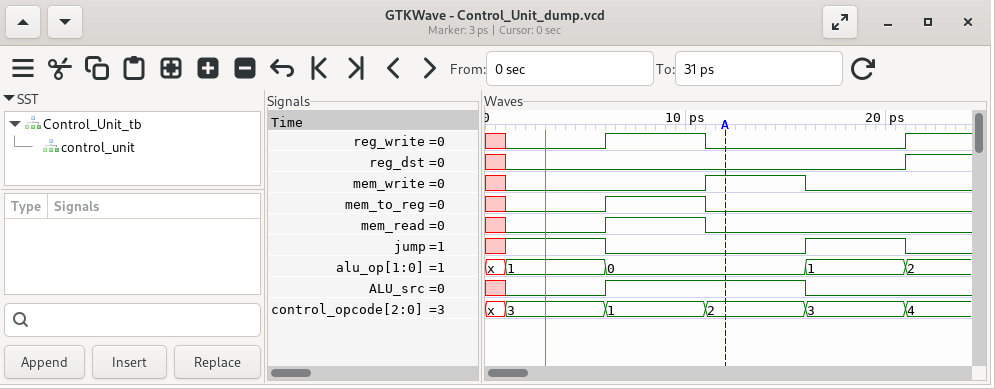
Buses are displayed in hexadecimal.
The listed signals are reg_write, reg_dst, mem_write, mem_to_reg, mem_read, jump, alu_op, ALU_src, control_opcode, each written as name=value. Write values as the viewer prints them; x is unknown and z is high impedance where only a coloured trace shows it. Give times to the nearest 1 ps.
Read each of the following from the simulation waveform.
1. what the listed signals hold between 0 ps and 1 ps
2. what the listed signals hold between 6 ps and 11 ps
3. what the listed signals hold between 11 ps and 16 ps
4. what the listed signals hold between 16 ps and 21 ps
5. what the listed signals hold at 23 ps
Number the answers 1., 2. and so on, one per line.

1. reg_write=x, reg_dst=x, mem_write=x, mem_to_reg=x, mem_read=x, jump=x, alu_op=x, ALU_src=x, control_opcode=x
2. reg_write=1, reg_dst=0, mem_write=0, mem_to_reg=1, mem_read=1, jump=0, alu_op=0, ALU_src=1, control_opcode=1
3. reg_write=0, reg_dst=0, mem_write=1, mem_to_reg=0, mem_read=0, jump=0, alu_op=0, ALU_src=1, control_opcode=2
4. reg_write=0, reg_dst=0, mem_write=0, mem_to_reg=0, mem_read=0, jump=1, alu_op=1, ALU_src=0, control_opcode=3
5. reg_write=1, reg_dst=1, mem_write=0, mem_to_reg=0, mem_read=0, jump=0, alu_op=2, ALU_src=0, control_opcode=4
